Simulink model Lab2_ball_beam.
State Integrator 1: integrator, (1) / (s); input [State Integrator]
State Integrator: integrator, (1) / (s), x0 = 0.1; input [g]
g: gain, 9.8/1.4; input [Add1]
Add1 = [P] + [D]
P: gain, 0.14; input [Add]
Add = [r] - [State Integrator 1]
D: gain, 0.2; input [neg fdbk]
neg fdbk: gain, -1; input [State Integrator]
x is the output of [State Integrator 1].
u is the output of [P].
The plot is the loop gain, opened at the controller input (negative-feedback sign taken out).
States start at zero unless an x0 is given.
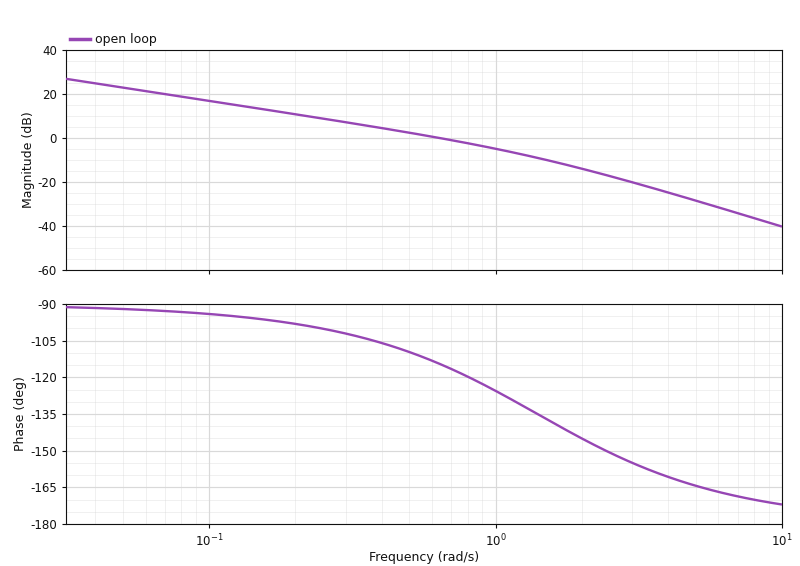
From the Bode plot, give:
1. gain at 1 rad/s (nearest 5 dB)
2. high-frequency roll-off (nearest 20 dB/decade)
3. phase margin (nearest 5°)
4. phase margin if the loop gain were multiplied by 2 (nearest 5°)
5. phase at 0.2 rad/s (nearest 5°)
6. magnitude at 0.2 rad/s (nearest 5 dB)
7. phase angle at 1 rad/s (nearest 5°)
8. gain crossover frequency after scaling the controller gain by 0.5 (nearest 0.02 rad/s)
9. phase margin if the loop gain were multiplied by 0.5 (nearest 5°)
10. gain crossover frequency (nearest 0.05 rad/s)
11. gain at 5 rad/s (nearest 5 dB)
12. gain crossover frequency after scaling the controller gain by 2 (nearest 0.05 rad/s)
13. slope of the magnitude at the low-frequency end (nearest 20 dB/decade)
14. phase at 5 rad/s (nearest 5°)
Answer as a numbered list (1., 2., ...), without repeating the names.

1. -5 dB
2. -40 dB/decade
3. 65°
4. 50°
5. -100°
6. 10 dB
7. -125°
8. 0.34 rad/s
9. 75°
10. 0.65 rad/s
11. -30 dB
12. 1.10 rad/s
13. -20 dB/decade
14. -165°
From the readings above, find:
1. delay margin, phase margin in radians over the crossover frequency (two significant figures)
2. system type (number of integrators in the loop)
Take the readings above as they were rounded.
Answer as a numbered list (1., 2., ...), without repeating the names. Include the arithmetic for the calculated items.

1. 65 × π / 180 / 0.65 = 1.7 s
2. 1
